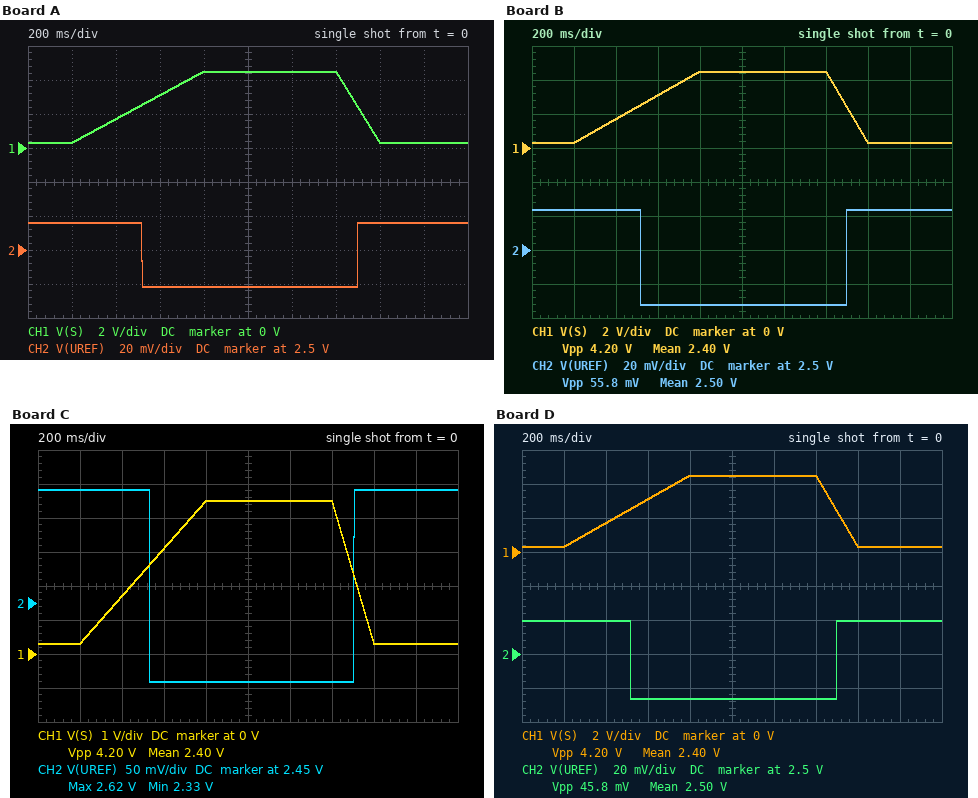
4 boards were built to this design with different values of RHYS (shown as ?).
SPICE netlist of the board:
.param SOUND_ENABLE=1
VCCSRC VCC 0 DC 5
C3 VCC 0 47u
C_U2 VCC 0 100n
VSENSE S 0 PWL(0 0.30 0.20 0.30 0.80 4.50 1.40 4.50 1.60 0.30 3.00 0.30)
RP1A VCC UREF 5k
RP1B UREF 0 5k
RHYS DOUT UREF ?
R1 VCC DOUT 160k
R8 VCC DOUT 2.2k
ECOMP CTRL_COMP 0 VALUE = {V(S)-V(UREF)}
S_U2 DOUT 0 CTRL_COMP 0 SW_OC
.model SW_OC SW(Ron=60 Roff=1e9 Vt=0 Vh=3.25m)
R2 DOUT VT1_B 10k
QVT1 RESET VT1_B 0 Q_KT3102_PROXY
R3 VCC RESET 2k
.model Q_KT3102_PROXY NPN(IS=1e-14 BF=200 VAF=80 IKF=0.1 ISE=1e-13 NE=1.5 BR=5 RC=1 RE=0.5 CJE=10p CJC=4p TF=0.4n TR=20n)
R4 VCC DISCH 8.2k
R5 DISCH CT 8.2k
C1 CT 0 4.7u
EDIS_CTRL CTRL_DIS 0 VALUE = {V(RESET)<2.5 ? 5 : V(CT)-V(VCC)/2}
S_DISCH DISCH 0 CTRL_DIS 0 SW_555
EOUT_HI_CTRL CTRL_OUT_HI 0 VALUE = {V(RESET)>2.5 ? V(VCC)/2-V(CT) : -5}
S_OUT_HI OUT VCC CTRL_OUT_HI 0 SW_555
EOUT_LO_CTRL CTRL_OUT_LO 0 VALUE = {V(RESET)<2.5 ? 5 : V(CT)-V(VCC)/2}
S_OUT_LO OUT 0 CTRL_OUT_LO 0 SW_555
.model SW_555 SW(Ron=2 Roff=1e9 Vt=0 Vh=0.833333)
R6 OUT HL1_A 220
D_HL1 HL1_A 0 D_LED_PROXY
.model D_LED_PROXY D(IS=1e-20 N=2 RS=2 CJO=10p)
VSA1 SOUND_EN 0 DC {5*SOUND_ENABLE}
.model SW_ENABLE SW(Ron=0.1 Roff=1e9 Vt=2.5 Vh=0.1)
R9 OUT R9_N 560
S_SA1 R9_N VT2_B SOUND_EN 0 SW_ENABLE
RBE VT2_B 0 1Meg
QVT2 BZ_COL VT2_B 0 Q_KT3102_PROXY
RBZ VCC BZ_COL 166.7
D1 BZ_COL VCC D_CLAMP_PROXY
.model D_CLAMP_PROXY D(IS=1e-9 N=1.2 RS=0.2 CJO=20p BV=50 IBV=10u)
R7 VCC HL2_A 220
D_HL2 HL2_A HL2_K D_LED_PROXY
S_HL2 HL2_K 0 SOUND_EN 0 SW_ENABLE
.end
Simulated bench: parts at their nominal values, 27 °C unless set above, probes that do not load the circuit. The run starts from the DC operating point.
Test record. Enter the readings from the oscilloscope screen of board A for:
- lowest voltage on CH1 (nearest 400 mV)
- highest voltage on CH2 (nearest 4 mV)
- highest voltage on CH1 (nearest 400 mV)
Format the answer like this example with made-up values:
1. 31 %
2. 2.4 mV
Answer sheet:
1. 400 mV
2. 2.516 V
3. 4.4 V
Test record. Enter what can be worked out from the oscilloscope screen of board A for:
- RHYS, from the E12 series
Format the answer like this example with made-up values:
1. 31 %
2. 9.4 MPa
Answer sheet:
1. 270 kΩ
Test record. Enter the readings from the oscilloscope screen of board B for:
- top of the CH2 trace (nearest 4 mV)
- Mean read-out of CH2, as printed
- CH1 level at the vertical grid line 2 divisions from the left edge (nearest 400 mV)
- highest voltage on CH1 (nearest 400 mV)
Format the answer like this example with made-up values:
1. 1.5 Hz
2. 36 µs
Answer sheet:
1. 2.524 V
2. 2.50 V
3. 1.6 V
4. 4.4 V
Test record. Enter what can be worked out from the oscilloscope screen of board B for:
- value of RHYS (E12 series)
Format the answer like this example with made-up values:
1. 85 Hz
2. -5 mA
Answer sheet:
1. 180 kΩ
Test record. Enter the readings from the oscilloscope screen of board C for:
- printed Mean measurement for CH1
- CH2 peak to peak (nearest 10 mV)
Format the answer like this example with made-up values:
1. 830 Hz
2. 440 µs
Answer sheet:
1. 2.40 V
2. 280 mV
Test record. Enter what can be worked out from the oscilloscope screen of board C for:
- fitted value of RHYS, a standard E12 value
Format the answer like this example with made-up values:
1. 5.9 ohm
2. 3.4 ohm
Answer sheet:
1. 33 kΩ
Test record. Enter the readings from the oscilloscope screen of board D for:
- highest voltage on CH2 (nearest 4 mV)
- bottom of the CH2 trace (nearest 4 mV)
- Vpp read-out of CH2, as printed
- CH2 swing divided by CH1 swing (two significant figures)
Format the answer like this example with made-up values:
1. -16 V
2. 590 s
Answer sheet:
1. 2.520 V
2. 2.472 V
3. 45.8 mV
4. 0.011
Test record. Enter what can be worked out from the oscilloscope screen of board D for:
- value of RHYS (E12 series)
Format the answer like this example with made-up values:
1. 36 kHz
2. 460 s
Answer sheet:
1. 220 kΩ
